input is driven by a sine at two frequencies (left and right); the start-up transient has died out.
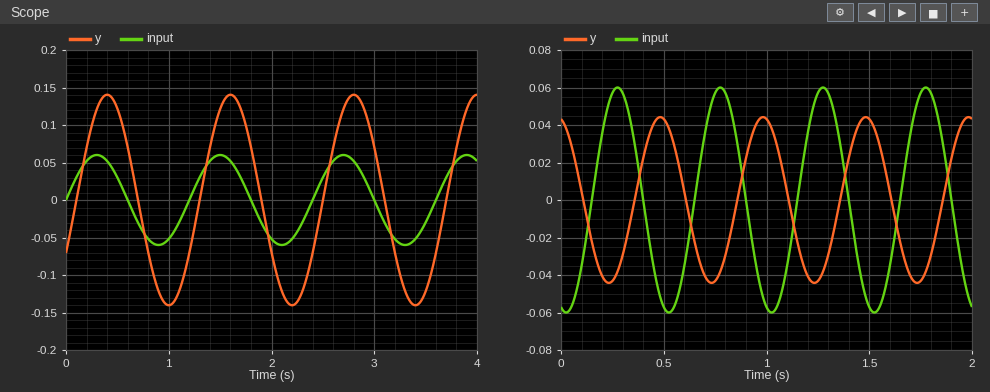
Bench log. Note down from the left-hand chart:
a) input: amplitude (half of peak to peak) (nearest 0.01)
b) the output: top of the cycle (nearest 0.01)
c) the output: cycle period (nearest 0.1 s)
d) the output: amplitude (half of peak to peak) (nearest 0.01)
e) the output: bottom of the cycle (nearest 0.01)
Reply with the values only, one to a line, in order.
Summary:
0.06
0.14
1.2 s
0.14
-0.14
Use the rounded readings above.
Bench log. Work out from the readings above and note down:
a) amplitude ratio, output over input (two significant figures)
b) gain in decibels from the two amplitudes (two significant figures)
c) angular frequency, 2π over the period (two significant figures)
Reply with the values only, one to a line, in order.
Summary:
2.3
7.4 dB
5.2 rad/s
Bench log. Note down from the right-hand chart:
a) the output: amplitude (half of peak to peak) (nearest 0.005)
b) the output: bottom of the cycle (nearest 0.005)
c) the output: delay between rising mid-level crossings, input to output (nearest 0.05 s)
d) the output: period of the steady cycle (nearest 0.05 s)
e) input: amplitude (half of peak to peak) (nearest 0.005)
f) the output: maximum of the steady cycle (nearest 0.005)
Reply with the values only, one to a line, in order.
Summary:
0.045
-0.045
0.20 s
0.50 s
0.060
0.045
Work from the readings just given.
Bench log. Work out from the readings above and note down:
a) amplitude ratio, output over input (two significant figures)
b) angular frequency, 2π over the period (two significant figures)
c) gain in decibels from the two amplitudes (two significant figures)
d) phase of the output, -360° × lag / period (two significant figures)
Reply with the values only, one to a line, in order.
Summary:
0.75
13 rad/s
-2.5 dB
-140°
